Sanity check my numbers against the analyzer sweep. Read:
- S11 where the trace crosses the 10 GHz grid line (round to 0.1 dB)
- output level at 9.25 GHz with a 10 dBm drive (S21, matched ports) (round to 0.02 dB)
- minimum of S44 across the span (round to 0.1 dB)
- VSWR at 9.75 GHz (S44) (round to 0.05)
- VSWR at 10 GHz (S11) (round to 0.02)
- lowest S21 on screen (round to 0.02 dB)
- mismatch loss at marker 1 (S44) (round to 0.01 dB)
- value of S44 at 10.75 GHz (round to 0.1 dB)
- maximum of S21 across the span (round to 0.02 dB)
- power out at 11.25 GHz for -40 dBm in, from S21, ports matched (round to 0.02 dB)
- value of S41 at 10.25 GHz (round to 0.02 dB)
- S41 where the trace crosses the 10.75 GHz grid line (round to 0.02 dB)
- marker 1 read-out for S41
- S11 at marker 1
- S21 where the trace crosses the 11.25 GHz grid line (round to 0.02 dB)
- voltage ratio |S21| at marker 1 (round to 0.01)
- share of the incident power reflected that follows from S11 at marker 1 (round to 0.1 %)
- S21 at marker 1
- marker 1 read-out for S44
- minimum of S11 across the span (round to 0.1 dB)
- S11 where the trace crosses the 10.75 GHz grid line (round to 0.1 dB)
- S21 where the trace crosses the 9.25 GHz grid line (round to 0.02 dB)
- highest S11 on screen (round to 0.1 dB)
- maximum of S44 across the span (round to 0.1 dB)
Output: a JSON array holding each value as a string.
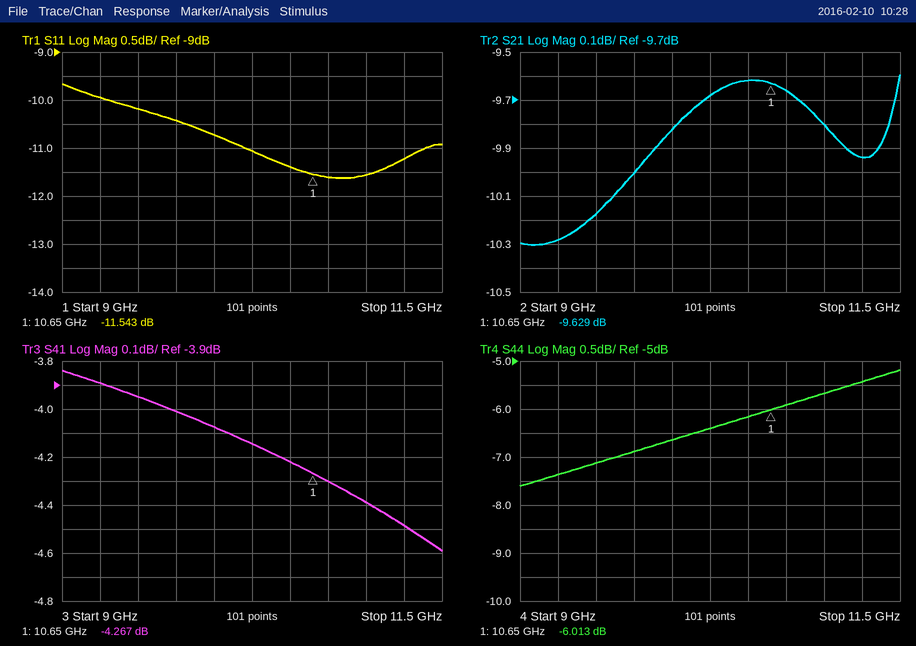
["-10.7 dB", "-0.28 dBm", "-7.6 dB", "2.65", "1.82", "-10.30 dB", "1.25 dB", "-5.9 dB", "-9.60 dB", "-49.94 dBm", "-4.14 dB", "-4.30 dB", "-4.267 dB", "-11.543 dB", "-9.94 dB", "0.33", "7.0 %", "-9.629 dB", "-6.013 dB", "-11.6 dB", "-11.6 dB", "-10.28 dB", "-9.7 dB", "-5.2 dB"]
